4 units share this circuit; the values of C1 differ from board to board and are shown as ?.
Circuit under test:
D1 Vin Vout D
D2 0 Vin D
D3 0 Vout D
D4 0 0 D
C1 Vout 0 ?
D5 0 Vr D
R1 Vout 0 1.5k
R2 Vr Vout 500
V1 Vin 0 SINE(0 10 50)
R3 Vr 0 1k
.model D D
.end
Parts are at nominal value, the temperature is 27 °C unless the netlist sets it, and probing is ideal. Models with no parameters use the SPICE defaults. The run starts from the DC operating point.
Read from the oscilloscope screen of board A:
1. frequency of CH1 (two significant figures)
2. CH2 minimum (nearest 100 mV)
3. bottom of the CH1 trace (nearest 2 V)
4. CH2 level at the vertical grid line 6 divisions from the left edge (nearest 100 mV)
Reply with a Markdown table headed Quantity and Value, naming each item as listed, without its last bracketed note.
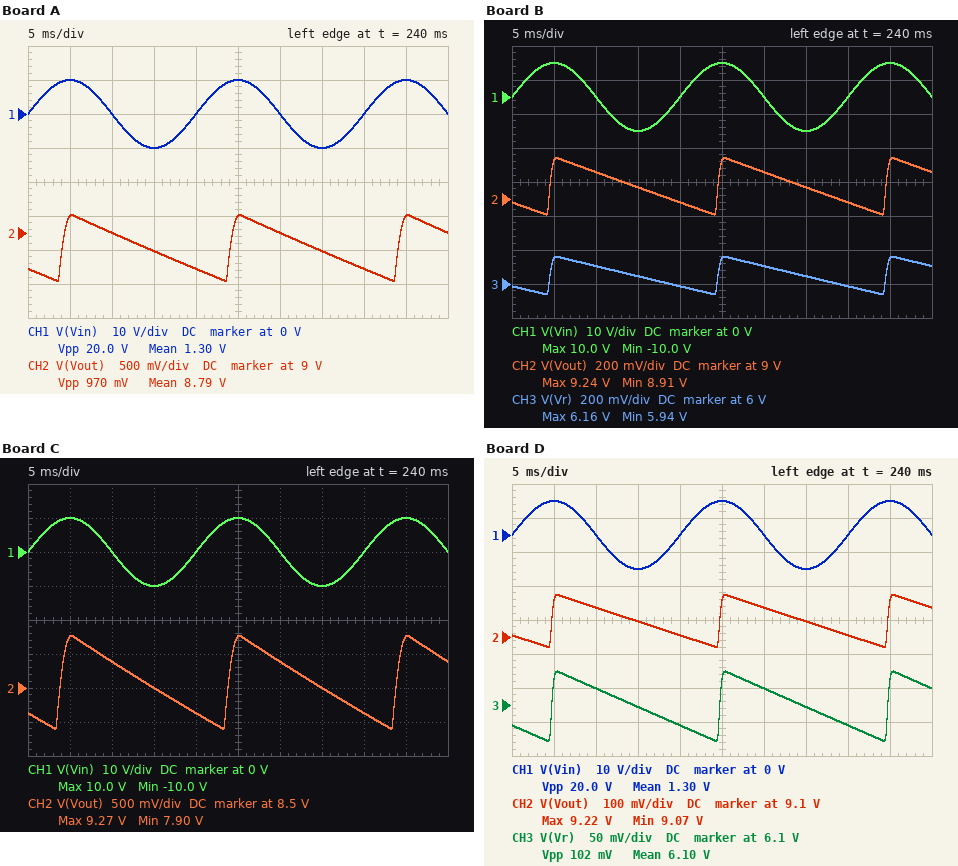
| Quantity | Value |
|---|---|
| frequency of CH1 | 50 Hz |
| CH2 minimum | 8.3 V |
| bottom of the CH1 trace | -10 V |
| CH2 level at the vertical grid line 6 divisions from the left edge | 9.0 V |
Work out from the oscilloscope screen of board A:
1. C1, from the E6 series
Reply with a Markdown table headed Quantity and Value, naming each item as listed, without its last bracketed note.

| Quantity | Value |
|---|---|
| C1, from the E6 series | 220 µF |
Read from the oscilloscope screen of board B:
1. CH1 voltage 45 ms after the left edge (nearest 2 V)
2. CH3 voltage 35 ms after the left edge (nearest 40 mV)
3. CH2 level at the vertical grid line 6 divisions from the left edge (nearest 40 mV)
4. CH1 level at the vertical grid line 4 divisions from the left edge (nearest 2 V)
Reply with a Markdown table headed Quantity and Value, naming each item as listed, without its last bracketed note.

| Quantity | Value |
|---|---|
| CH1 voltage 45 ms after the left edge | 10 V |
| CH3 voltage 35 ms after the left edge | 6.04 V |
| CH2 level at the vertical grid line 6 divisions from the left edge | 9.16 V |
| CH1 level at the vertical grid line 4 divisions from the left edge | 0 V |
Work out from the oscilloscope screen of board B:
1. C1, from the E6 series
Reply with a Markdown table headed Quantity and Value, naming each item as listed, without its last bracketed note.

| Quantity | Value |
|---|---|
| C1, from the E6 series | 680 µF |
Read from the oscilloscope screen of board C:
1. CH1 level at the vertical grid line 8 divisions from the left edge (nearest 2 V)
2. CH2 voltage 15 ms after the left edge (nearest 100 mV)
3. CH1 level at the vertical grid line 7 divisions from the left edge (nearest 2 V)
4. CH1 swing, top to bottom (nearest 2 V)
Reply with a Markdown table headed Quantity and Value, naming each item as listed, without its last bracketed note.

| Quantity | Value |
|---|---|
| CH1 level at the vertical grid line 8 divisions from the left edge | 0 V |
| CH2 voltage 15 ms after the left edge | 8.5 V |
| CH1 level at the vertical grid line 7 divisions from the left edge | -10 V |
| CH1 swing, top to bottom | 20 V |
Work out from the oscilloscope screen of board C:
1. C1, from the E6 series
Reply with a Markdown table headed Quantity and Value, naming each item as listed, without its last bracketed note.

| Quantity | Value |
|---|---|
| C1, from the E6 series | 150 µF |
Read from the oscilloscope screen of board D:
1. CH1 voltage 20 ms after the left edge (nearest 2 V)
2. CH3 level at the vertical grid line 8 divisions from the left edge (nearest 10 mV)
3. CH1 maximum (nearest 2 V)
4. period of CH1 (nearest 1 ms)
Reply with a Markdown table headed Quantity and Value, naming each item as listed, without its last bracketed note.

| Quantity | Value |
|---|---|
| CH1 voltage 20 ms after the left edge | 0 V |
| CH3 level at the vertical grid line 8 divisions from the left edge | 6.07 V |
| CH1 maximum | 10 V |
| period of CH1 | 20 ms |
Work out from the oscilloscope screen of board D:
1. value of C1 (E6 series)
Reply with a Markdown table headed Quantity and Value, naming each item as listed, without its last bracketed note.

| Quantity | Value |
|---|---|
| value of C1 | 1.5 mF |
